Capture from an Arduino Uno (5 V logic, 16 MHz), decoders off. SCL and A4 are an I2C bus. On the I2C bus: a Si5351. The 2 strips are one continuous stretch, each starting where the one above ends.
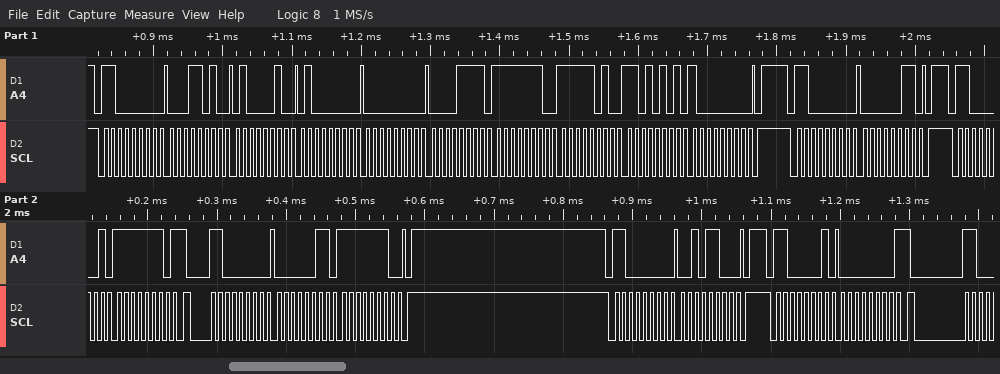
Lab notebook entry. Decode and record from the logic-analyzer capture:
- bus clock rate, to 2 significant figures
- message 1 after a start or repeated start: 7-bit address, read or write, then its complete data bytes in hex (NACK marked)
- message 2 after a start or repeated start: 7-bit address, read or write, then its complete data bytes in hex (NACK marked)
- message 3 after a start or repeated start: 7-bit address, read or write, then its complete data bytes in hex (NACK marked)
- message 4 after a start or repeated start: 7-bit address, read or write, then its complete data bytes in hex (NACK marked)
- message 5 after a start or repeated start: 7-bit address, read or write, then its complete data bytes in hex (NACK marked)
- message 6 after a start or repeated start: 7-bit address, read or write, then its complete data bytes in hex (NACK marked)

100 kHz
0x60 write: 1A 42 40 00 0F FE FA D5 80
0x60 write: 03
0x60 read: FE NACK
0x60 write: 03 FE
0x60 write: 2C
0x60 read: 00 NACK
